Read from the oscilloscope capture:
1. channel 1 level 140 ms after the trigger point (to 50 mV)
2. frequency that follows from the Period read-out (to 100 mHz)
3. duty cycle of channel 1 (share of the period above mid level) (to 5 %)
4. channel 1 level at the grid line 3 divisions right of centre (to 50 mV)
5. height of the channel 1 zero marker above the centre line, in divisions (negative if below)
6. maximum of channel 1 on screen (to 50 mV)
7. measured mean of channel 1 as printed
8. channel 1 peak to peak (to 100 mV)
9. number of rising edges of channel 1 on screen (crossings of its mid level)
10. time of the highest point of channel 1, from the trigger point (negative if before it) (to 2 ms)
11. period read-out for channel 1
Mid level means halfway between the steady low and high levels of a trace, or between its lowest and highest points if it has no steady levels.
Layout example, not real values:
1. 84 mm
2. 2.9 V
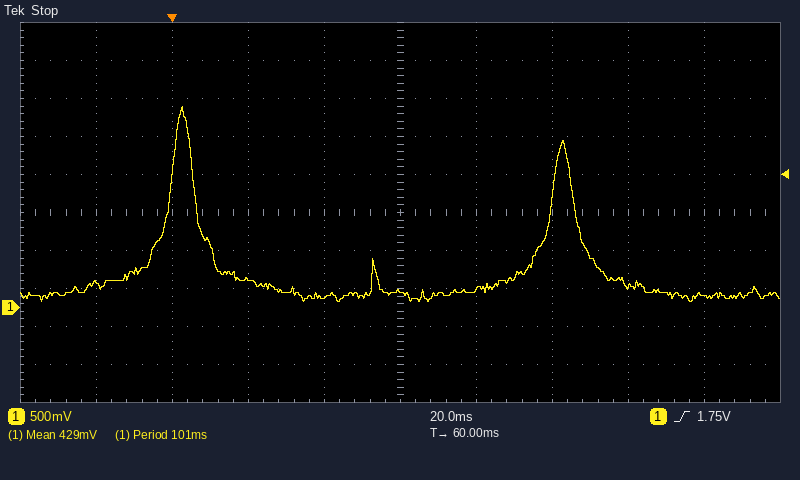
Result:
1. 150 mV
2. 9.9 Hz
3. 5 %
4. 300 mV
5. -2.5 div
6. 2.65 V
7. 429 mV
8. 2.60 V
9. 2
10. +2 ms
11. 101 ms
